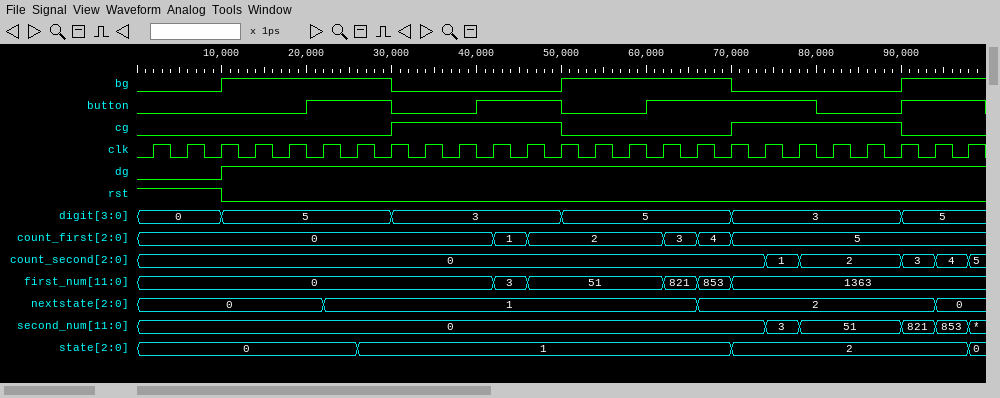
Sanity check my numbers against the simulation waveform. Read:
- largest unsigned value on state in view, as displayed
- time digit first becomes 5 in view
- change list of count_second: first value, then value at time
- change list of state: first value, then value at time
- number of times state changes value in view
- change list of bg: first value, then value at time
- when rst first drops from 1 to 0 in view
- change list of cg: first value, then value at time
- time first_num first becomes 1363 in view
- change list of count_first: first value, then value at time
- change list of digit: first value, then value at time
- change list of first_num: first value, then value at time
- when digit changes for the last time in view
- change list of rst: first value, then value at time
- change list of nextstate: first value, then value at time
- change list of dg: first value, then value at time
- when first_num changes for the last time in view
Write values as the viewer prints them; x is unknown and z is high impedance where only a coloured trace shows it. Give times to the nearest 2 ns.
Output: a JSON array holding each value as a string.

["2", "10 ns", "0, 1 at 74 ns, 2 at 78 ns, 3 at 90 ns, 4 at 94 ns, 5 at 98 ns", "0, 1 at 26 ns, 2 at 70 ns, 0 at 98 ns", "3", "0, 1 at 10 ns, 0 at 30 ns, 1 at 50 ns, 0 at 70 ns, 1 at 90 ns", "10 ns", "0, 1 at 30 ns, 0 at 50 ns, 1 at 70 ns, 0 at 90 ns", "70 ns", "0, 1 at 42 ns, 2 at 46 ns, 3 at 62 ns, 4 at 66 ns, 5 at 70 ns", "0, 5 at 10 ns, 3 at 30 ns, 5 at 50 ns, 3 at 70 ns, 5 at 90 ns", "0, 3 at 42 ns, 51 at 46 ns, 821 at 62 ns, 853 at 66 ns, 1363 at 70 ns", "90 ns", "1, 0 at 10 ns", "0, 1 at 22 ns, 2 at 66 ns, 0 at 94 ns", "0, 1 at 10 ns", "70 ns"]
